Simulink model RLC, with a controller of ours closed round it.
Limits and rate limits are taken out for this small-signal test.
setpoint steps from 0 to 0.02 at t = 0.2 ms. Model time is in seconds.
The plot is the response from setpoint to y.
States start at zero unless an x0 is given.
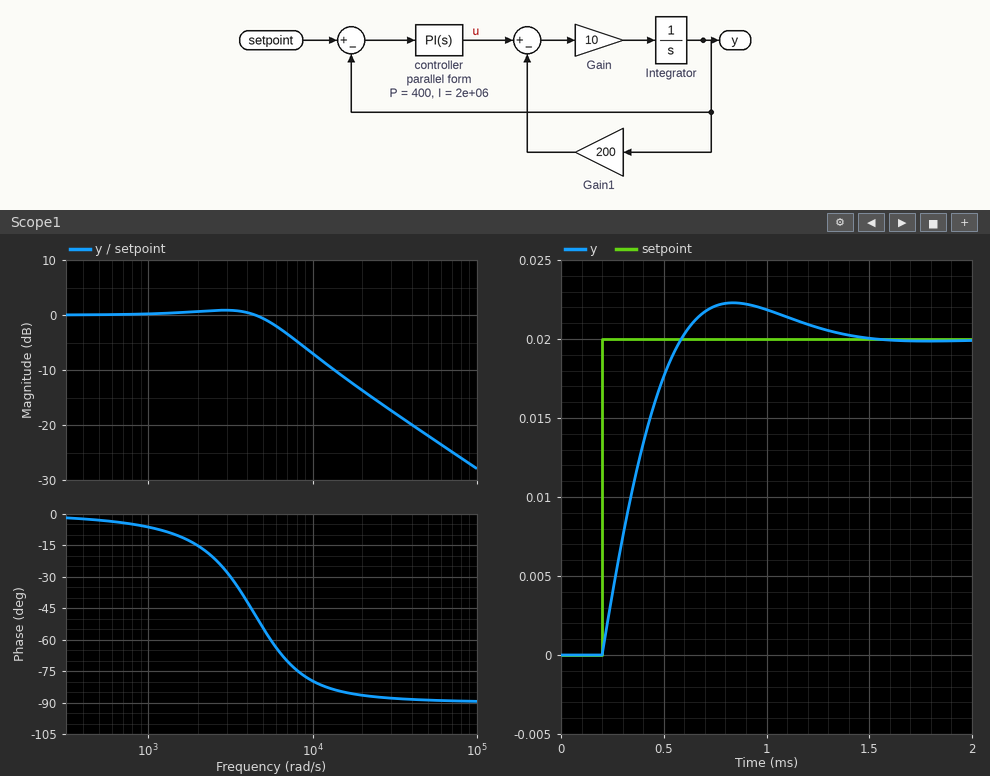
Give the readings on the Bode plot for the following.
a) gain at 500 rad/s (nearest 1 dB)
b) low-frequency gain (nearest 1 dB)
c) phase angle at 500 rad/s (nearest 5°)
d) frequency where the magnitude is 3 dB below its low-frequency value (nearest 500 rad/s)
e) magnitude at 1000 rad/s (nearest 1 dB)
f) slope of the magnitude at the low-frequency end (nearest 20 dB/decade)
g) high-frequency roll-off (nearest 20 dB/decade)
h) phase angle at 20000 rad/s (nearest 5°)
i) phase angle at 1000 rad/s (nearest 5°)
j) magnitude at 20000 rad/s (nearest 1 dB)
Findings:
0 dB
0 dB
-5°
6500 rad/s
0 dB
0 dB/decade
-20 dB/decade
-85°
-5°
-14 dB
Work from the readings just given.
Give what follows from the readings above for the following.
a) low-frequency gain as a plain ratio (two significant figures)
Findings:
1.0
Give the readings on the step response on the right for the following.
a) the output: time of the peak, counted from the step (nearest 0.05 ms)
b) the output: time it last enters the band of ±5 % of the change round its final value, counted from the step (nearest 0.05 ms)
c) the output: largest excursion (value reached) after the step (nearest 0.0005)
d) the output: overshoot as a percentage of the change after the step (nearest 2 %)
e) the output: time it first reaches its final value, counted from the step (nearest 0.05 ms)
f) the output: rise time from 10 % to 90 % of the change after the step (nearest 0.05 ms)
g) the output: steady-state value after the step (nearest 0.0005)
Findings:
0.65 ms
1.00 ms
0.0225
12 %
0.40 ms
0.30 ms
0.0200
